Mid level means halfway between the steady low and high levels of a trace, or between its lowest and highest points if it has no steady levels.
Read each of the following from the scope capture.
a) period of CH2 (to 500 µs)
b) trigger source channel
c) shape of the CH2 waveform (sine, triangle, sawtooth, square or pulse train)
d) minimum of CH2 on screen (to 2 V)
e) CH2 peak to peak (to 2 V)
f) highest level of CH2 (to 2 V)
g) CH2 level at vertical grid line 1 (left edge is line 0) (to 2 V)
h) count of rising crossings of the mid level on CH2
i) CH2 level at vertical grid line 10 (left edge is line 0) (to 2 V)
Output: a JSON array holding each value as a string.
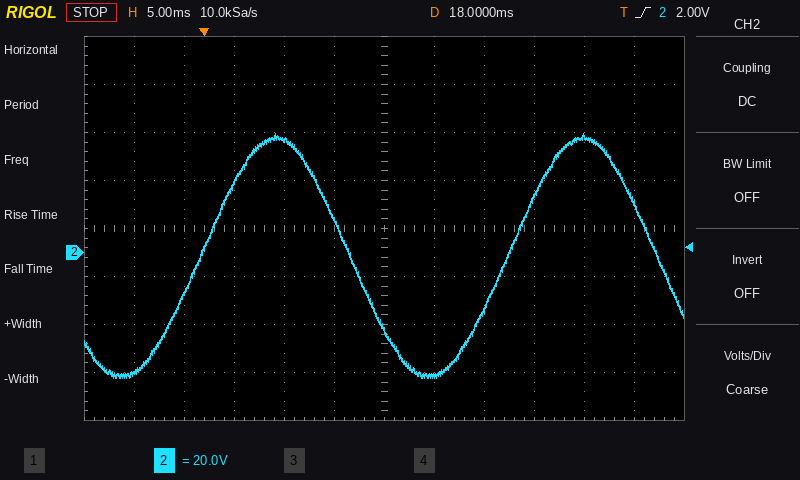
["30.5 ms", "CH2", "sine", "-52 V", "102 V", "50 V", "-50 V", "2", "48 V"]
